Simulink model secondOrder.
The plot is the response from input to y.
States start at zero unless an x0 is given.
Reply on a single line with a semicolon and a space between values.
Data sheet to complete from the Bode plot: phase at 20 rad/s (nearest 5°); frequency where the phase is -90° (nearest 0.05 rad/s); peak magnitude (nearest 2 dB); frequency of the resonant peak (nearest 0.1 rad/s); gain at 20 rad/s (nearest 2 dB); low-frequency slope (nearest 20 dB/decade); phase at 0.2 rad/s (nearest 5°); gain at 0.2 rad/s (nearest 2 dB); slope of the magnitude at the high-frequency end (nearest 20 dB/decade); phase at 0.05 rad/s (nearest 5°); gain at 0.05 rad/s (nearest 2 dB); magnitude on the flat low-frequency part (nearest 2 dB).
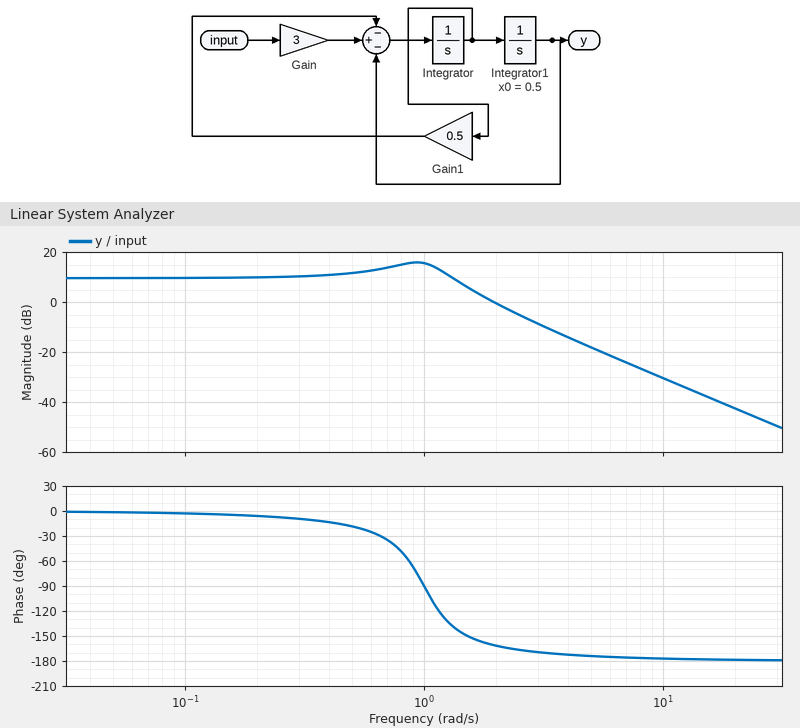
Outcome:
-180°; 1.00 rad/s; 16 dB; 0.9 rad/s; -42 dB; 0 dB/decade; -5°; 10 dB; -40 dB/decade; 0°; 10 dB; 10 dB
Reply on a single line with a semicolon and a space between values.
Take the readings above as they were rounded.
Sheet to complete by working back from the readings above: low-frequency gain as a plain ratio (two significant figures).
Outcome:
3.2
